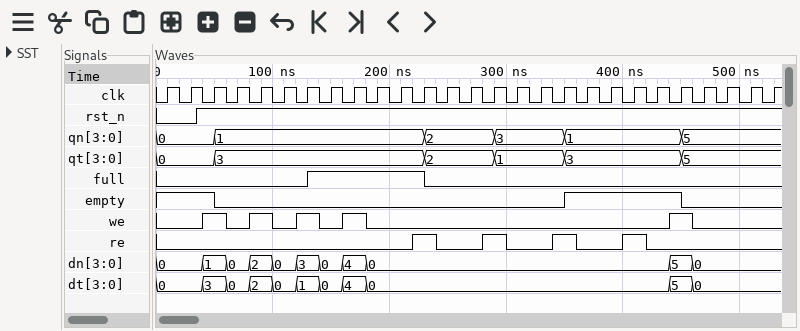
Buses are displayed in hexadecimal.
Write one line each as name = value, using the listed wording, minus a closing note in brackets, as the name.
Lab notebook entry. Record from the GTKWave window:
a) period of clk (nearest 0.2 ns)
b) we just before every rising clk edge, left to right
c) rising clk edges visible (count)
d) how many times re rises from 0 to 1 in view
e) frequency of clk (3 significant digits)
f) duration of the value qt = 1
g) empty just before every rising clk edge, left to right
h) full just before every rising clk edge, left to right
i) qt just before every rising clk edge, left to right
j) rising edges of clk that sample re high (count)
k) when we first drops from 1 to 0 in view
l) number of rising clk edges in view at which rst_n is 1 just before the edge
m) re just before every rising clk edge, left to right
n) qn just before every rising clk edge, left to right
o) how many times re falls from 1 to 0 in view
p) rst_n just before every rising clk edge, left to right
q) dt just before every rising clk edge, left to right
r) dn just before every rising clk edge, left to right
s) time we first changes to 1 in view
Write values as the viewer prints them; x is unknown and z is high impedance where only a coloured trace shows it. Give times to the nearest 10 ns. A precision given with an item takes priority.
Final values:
period of clk = 20 ns
we just before every rising clk edge, left to right = 0 0 1 0 1 0 1 0 1 0 0 0 0 0 0 0 0 0 0 0 0 0 1 0 0 0 0
rising clk edges visible = 27
how many times re rises from 0 to 1 in view = 4
frequency of clk = 50.0 MHz
duration of the value qt = 1 = 60 ns
empty just before every rising clk edge, left to right = 1 1 1 0 0 0 0 0 0 0 0 0 0 0 0 0 0 0 1 1 1 1 1 0 0 0 0
full just before every rising clk edge, left to right = 0 0 0 0 0 0 0 1 1 1 1 1 0 0 0 0 0 0 0 0 0 0 0 0 0 0 0
qt just before every rising clk edge, left to right = 0, 0, 0, 3, 3, 3, 3, 3, 3, 3, 3, 3, 2, 2, 2, 1, 1, 1, 3, 3, 3, 3, 3, 5, 5, 5, 5
rising edges of clk that sample re high = 4
when we first drops from 1 to 0 in view = 60 ns
number of rising clk edges in view at which rst_n is 1 just before the edge = 25
re just before every rising clk edge, left to right = 0 0 0 0 0 0 0 0 0 0 0 1 0 0 1 0 0 1 0 0 1 0 0 0 0 0 0
qn just before every rising clk edge, left to right = 0, 0, 0, 1, 1, 1, 1, 1, 1, 1, 1, 1, 2, 2, 2, 3, 3, 3, 1, 1, 1, 1, 1, 5, 5, 5, 5
how many times re falls from 1 to 0 in view = 4
rst_n just before every rising clk edge, left to right = 0 0 1 1 1 1 1 1 1 1 1 1 1 1 1 1 1 1 1 1 1 1 1 1 1 1 1
dt just before every rising clk edge, left to right = 0, 0, 3, 0, 2, 0, 1, 0, 4, 0, 0, 0, 0, 0, 0, 0, 0, 0, 0, 0, 0, 0, 5, 0, 0, 0, 0
dn just before every rising clk edge, left to right = 0, 0, 1, 0, 2, 0, 3, 0, 4, 0, 0, 0, 0, 0, 0, 0, 0, 0, 0, 0, 0, 0, 5, 0, 0, 0, 0
time we first changes to 1 in view = 40 ns
